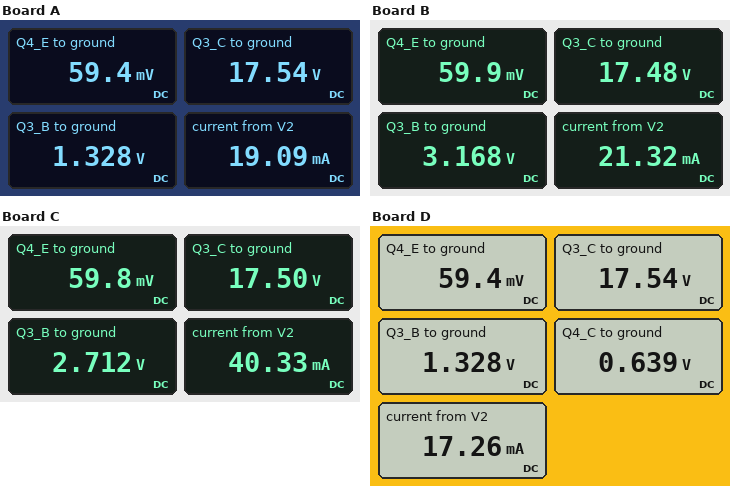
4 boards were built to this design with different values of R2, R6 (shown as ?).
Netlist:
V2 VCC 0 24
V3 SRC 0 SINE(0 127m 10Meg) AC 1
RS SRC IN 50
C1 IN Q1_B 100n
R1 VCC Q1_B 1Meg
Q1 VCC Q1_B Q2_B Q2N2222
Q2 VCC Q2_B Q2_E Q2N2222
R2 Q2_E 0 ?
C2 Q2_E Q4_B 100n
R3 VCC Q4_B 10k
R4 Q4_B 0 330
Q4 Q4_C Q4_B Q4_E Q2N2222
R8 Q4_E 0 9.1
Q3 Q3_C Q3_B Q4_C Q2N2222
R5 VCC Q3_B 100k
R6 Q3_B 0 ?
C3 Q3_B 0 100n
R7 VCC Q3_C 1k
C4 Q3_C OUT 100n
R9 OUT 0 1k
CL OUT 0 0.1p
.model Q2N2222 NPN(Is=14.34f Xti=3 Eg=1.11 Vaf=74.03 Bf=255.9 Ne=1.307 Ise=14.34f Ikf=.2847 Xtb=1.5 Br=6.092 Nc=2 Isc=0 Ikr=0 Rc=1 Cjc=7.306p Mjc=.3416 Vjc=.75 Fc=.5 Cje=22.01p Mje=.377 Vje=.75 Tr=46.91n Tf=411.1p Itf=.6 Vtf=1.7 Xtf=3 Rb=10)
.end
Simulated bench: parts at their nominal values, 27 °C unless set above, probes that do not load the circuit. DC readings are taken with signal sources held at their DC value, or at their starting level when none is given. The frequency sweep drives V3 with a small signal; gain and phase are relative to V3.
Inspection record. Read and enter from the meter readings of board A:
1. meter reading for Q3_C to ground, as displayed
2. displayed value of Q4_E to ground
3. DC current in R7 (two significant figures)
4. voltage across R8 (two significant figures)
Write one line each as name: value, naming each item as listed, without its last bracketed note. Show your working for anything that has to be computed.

meter reading for Q3_C to ground, as displayed: 17.54 V
displayed value of Q4_E to ground: 59.4 mV
DC current in R7: (24 V - 17.54 V) / 1 kΩ = 6.5 mA
voltage across R8: 59.4 mV = 59 mV
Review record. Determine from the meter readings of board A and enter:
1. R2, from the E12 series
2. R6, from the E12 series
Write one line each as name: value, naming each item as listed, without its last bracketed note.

R2, from the E12 series: 2.2 kΩ
R6, from the E12 series: 6.8 kΩ
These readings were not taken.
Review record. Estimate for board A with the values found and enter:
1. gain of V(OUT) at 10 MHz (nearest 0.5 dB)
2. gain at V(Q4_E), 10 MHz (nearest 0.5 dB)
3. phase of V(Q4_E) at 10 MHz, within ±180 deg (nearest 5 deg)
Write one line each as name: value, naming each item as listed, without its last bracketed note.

gain of V(OUT) at 10 MHz: 30.5 dB
gain at V(Q4_E), 10 MHz: -4.0 dB
phase of V(Q4_E) at 10 MHz, within ±180 deg: -10 deg
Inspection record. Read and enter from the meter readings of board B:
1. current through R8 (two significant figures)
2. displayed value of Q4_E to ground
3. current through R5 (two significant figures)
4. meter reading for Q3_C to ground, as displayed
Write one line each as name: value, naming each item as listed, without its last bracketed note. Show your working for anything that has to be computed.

current through R8: (59.9 mV) / 9.1 Ω = 6.6 mA
displayed value of Q4_E to ground: 59.9 mV
current through R5: (24 V - 3.168 V) / 100 kΩ = 210 µA
meter reading for Q3_C to ground, as displayed: 17.48 V
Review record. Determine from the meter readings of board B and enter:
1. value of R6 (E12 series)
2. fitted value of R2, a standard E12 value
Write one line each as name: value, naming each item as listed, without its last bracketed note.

value of R6: 18 kΩ
fitted value of R2, a standard E12 value: 1.8 kΩ
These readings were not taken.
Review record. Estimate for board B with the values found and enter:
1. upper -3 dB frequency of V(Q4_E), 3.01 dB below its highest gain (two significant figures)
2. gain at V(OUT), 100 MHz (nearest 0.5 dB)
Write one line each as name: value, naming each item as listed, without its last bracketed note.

upper -3 dB frequency of V(Q4_E), 3.01 dB below its highest gain: 77 MHz
gain at V(OUT), 100 MHz: 23.0 dB
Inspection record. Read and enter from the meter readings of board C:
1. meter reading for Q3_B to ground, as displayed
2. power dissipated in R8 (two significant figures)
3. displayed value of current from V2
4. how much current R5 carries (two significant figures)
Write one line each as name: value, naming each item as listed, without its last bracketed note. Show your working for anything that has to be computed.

meter reading for Q3_B to ground, as displayed: 2.712 V
power dissipated in R8: (59.8 mV)^2 / 9.1 Ω = 390 µW
displayed value of current from V2: 40.33 mA
how much current R5 carries: (24 V - 2.712 V) / 100 kΩ = 210 µA
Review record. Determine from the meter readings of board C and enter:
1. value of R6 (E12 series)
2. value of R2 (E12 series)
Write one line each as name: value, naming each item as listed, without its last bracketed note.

value of R6: 15 kΩ
value of R2: 680 Ω
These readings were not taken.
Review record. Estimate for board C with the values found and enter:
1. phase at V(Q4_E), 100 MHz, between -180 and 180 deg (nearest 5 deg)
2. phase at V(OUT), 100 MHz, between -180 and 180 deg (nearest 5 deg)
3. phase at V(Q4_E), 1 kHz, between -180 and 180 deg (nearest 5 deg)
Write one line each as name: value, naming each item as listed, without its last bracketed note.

phase at V(Q4_E), 100 MHz, between -180 and 180 deg: -65 deg
phase at V(OUT), 100 MHz, between -180 and 180 deg: 30 deg
phase at V(Q4_E), 1 kHz, between -180 and 180 deg: 80 deg
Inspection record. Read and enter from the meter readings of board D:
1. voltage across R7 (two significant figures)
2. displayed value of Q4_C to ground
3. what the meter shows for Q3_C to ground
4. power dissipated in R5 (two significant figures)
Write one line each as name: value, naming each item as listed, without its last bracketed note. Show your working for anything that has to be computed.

voltage across R7: 24 V - 17.54 V = 6.5 V
displayed value of Q4_C to ground: 0.639 V
what the meter shows for Q3_C to ground: 17.54 V
power dissipated in R5: (24 V - 1.328 V)^2 / 100 kΩ = 5.1 mW
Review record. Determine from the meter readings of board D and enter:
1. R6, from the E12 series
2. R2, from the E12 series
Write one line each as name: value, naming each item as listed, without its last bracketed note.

R6, from the E12 series: 6.8 kΩ
R2, from the E12 series: 2.7 kΩ
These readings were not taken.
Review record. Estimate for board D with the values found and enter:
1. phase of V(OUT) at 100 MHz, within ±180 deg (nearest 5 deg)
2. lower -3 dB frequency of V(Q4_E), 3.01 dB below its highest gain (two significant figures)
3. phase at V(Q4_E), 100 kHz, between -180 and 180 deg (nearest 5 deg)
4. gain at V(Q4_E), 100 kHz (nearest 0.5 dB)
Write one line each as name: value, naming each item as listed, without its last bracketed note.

phase of V(OUT) at 100 MHz, within ±180 deg: 25 deg
lower -3 dB frequency of V(Q4_E), 3.01 dB below its highest gain: 5.5 kHz
phase at V(Q4_E), 100 kHz, between -180 and 180 deg: 5 deg
gain at V(Q4_E), 100 kHz: -3.5 dB
